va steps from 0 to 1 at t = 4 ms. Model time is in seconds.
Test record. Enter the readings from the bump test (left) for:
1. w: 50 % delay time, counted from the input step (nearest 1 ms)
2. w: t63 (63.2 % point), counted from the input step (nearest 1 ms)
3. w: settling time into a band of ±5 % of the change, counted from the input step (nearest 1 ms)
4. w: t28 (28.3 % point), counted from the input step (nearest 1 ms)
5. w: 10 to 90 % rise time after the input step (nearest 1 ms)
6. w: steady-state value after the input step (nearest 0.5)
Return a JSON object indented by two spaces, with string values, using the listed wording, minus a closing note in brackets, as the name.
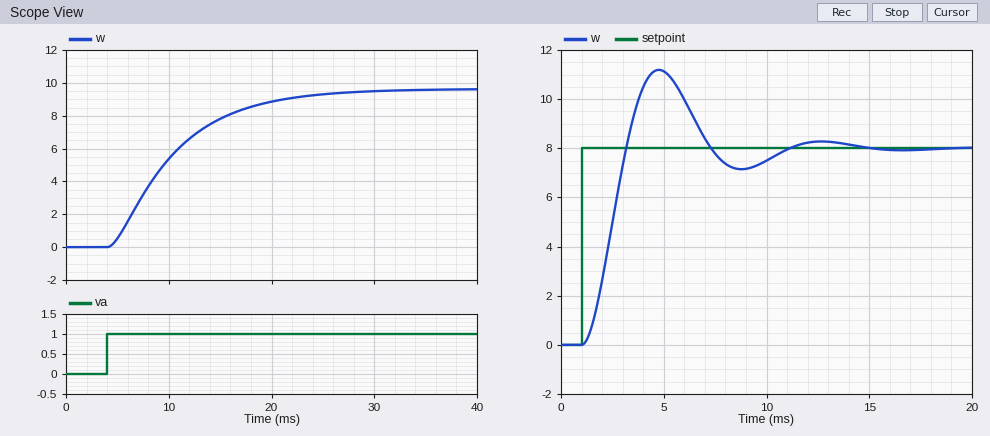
{
  "w: 50 % delay time, counted from the input step": "5 ms",
  "w: t63 (63.2 % point), counted from the input step": "7 ms",
  "w: settling time into a band of ±5 % of the change, counted from the input step": "19 ms",
  "w: t28 (28.3 % point), counted from the input step": "3 ms",
  "w: 10 to 90 % rise time after the input step": "13 ms",
  "w: steady-state value after the input step": "9.5"
}
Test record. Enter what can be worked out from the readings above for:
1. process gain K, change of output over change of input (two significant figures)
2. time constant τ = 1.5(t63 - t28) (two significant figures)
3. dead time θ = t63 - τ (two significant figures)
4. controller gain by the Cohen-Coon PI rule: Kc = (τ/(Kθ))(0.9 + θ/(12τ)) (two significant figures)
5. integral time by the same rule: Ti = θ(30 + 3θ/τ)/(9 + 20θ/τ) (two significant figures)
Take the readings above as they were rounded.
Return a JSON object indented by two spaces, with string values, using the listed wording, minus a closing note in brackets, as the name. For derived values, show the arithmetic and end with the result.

{
  "process gain K, change of output over change of input": "(9.5 - 0) / 1 = 9.5",
  "time constant τ = 1.5(t63 - t28)": "1.5 × (7 - 3) = 6.0 ms",
  "dead time θ = t63 - τ": "7 - 6 = 1.0 ms",
  "controller gain by the Cohen-Coon PI rule: Kc = (τ/(Kθ))(0.9 + θ/(12τ))": "6 / (9.5 × 1) × (0.9 + 1 / (12 × 6)) = 0.58",
  "integral time by the same rule: Ti = θ(30 + 3θ/τ)/(9 + 20θ/τ)": "1 × (30 + 3 × 1 / 6) / (9 + 20 × 1 / 6) = 2.5 ms"
}
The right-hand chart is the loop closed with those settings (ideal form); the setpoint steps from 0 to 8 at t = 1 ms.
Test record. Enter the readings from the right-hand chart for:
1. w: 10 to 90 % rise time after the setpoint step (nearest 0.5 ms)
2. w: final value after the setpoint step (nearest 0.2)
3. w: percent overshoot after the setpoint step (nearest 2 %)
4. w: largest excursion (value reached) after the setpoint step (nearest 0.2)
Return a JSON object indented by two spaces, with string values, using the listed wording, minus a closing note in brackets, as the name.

{
  "w: 10 to 90 % rise time after the setpoint step": "1.5 ms",
  "w: final value after the setpoint step": "8.0",
  "w: percent overshoot after the setpoint step": "40 %",
  "w: largest excursion (value reached) after the setpoint step": "11.2"
}
